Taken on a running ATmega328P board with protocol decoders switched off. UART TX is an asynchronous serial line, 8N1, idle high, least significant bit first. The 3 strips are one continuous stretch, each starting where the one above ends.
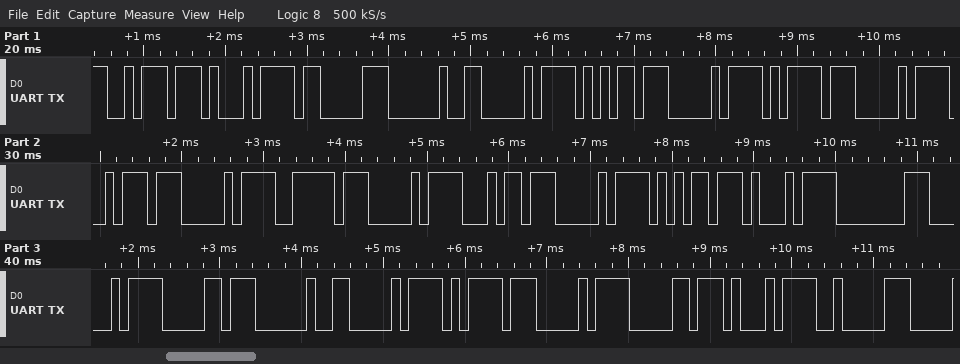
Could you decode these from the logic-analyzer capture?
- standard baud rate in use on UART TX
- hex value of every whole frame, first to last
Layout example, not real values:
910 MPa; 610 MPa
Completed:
9600 baud; 0xBA 0xD1 0x83 0x20 0xD0 0xB5 0xD0 0xBD 0xD0 0xBA 0xD0 0xBE 0xD0 0xB4 0xD0 0xB5 0xD1 0x80 0xD0 0xB0 0x20 0xD0 0xBD 0xD0 0xB0 0xD1 0x82
